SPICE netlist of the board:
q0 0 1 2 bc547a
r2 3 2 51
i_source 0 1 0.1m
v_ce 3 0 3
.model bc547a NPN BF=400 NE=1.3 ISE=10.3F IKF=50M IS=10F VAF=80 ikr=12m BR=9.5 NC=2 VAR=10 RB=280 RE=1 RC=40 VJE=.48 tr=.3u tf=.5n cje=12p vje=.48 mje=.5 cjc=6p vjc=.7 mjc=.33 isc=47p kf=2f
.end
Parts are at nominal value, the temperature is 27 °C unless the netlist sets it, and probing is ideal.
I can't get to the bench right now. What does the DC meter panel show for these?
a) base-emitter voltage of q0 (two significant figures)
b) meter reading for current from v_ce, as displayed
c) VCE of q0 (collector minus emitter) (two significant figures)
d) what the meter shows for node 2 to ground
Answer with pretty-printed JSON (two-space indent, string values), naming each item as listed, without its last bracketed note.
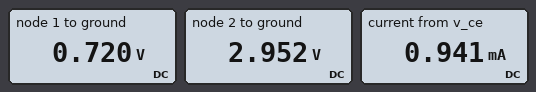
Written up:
{
  "base-emitter voltage of q0": "-2.2 V",
  "meter reading for current from v_ce, as displayed": "0.941 mA",
  "VCE of q0 (collector minus emitter)": "-3.0 V",
  "what the meter shows for node 2 to ground": "2.952 V"
}
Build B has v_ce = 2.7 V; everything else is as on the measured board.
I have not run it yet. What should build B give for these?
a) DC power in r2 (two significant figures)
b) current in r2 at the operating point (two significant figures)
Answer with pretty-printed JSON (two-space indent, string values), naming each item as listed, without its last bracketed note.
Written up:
{
  "DC power in r2": "43 µW",
  "current in r2 at the operating point": "920 µA"
}
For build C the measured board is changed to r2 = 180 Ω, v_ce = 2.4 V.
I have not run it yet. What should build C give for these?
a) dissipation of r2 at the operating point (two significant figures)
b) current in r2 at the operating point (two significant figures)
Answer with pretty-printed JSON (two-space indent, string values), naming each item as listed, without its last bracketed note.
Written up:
{
  "dissipation of r2 at the operating point": "140 µW",
  "current in r2 at the operating point": "890 µA"
}
